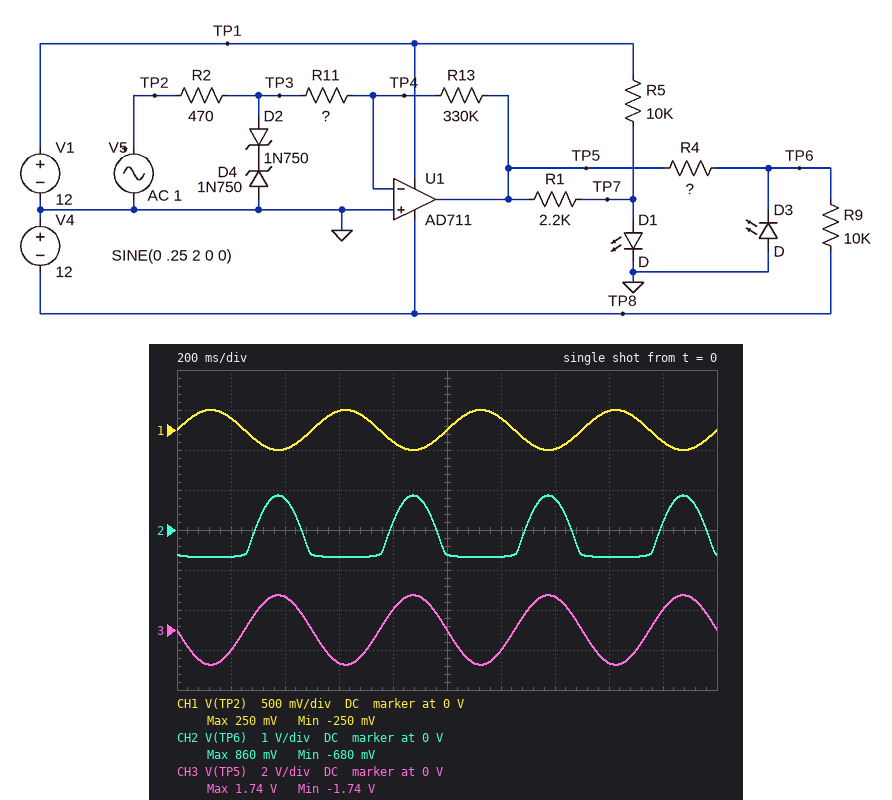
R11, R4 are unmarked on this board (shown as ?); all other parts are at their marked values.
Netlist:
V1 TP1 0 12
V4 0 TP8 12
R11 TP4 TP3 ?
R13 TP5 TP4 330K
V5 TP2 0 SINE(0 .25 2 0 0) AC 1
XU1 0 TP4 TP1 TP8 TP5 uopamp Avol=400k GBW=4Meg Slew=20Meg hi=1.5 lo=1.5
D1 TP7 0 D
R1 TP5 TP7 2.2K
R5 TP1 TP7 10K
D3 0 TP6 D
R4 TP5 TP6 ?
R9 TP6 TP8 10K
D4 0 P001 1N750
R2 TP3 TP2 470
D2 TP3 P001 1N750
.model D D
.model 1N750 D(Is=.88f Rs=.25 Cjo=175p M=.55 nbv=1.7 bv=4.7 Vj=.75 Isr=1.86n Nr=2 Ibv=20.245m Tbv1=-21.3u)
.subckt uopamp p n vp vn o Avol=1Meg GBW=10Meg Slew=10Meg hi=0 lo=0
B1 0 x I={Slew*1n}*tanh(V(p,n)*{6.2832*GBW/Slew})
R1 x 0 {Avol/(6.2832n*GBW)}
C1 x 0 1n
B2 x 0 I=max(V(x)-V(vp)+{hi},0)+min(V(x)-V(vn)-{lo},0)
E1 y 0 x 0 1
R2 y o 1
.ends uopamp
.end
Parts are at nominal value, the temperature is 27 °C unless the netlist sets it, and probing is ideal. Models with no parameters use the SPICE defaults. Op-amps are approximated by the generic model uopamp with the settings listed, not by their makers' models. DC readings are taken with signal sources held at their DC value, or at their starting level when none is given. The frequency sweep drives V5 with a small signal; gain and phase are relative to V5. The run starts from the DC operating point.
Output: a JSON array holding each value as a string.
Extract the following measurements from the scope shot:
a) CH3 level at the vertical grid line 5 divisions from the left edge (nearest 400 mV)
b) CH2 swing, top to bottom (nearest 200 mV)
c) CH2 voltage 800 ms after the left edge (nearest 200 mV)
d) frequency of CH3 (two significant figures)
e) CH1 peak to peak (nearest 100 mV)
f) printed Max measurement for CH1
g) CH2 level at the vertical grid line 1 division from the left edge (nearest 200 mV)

["0 V", "1.6 V", "200 mV", "2.0 Hz", "500 mV", "250 mV", "-600 mV"]
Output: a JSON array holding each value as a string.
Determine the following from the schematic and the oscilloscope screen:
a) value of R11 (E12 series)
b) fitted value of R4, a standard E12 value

["47 kΩ", "680 Ω"]
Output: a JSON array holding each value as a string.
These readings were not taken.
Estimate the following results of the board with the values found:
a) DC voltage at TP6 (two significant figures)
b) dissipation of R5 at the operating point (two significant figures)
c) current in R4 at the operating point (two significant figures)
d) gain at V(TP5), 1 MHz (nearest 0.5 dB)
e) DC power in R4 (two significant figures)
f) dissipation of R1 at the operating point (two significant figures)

["-620 mV", "13 mW", "910 µA", "9.5 dB", "560 µW", "190 µW"]
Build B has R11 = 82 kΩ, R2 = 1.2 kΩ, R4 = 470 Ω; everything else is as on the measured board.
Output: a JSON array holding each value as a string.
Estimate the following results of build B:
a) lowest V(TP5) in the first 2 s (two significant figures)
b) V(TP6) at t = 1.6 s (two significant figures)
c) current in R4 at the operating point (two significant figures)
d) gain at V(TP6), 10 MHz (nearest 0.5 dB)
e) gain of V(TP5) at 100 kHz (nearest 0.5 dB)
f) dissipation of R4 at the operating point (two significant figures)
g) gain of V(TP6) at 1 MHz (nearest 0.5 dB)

["-990 mV", "-670 mV", "1.1 mA", "-28.0 dB", "12.0 dB", "610 µW", "4.5 dB"]
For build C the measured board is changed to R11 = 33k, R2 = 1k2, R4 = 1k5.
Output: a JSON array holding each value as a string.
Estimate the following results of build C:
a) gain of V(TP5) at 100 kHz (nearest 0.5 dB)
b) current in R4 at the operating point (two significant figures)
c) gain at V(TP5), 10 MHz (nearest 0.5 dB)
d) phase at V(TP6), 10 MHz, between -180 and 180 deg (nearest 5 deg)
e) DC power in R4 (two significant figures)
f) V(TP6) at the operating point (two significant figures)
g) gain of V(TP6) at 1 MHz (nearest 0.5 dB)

["19.5 dB", "430 µA", "-25.5 dB", "10 deg", "280 µW", "-650 mV", "-23.5 dB"]
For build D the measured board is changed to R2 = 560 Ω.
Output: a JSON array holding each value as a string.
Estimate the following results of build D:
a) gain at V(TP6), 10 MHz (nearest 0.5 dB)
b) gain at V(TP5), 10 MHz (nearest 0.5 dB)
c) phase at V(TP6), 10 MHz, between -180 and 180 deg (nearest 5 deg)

["-36.5 dB", "-19.5 dB", "20 deg"]
